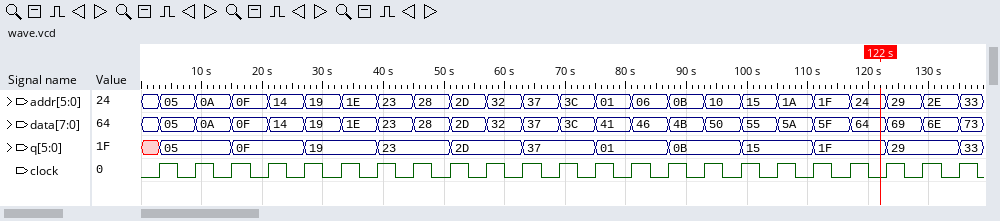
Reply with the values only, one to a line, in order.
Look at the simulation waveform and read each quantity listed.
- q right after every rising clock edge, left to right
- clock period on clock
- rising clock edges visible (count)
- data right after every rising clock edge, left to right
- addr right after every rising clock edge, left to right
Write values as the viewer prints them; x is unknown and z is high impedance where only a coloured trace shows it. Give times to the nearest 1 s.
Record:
05, 05, 0F, 0F, 19, 19, 23, 23, 2D, 2D, 37, 37, 01, 01, 0B, 0B, 15, 15, 1F, 1F, 29, 29, 33
6 s
23
05, 0A, 0F, 14, 19, 1E, 23, 28, 2D, 32, 37, 3C, 41, 46, 4B, 50, 55, 5A, 5F, 64, 69, 6E, 73
05, 0A, 0F, 14, 19, 1E, 23, 28, 2D, 32, 37, 3C, 01, 06, 0B, 10, 15, 1A, 1F, 24, 29, 2E, 33
